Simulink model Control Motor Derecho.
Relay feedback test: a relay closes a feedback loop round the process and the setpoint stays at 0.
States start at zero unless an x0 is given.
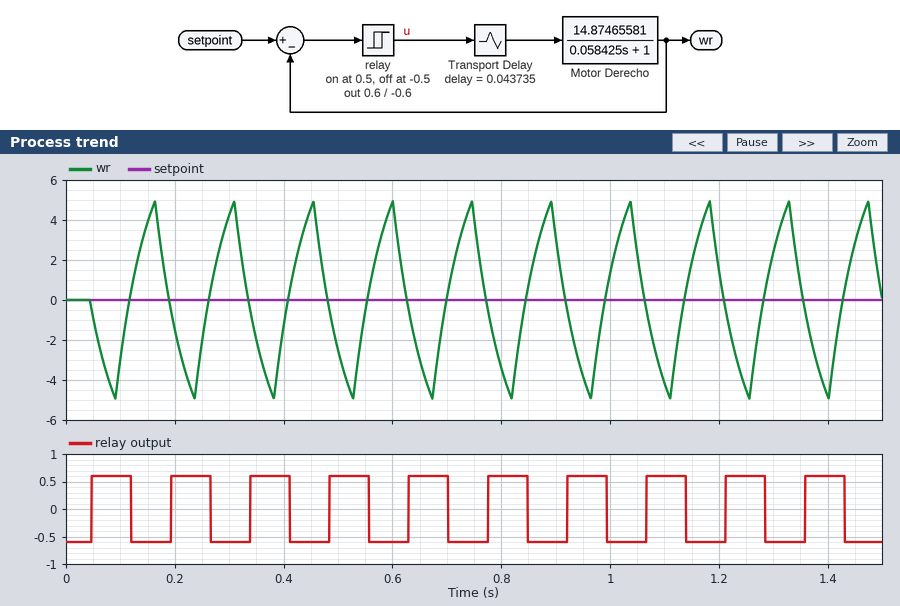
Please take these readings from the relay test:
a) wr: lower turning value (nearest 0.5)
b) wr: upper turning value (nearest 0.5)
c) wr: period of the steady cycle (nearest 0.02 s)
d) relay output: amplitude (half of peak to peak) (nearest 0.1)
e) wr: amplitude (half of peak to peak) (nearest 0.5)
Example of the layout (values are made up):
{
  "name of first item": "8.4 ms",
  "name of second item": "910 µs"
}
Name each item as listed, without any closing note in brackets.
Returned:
{
  "wr: lower turning value": "-5.0",
  "wr: upper turning value": "5.0",
  "wr: period of the steady cycle": "0.14 s",
  "relay output: amplitude (half of peak to peak)": "0.6",
  "wr: amplitude (half of peak to peak)": "5.0"
}
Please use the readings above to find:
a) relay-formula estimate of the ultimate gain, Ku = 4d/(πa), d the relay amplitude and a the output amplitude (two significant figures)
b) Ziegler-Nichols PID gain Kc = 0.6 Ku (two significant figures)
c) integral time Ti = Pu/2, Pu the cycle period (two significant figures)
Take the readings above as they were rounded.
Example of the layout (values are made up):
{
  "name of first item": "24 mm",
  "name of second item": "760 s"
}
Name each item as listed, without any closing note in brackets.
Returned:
{
  "relay-formula estimate of the ultimate gain, Ku = 4d/(πa), d the relay amplitude and a the output amplitude": "0.15",
  "Ziegler-Nichols PID gain Kc = 0.6 Ku": "0.090",
  "integral time Ti = Pu/2, Pu the cycle period": "0.070 s"
}
